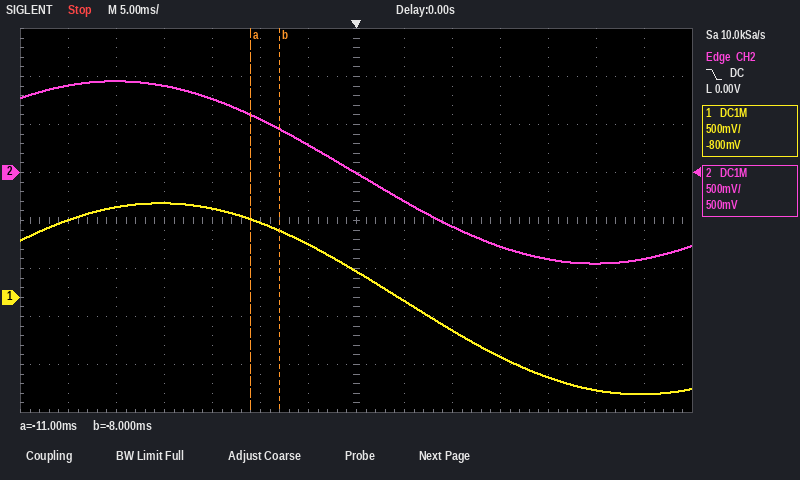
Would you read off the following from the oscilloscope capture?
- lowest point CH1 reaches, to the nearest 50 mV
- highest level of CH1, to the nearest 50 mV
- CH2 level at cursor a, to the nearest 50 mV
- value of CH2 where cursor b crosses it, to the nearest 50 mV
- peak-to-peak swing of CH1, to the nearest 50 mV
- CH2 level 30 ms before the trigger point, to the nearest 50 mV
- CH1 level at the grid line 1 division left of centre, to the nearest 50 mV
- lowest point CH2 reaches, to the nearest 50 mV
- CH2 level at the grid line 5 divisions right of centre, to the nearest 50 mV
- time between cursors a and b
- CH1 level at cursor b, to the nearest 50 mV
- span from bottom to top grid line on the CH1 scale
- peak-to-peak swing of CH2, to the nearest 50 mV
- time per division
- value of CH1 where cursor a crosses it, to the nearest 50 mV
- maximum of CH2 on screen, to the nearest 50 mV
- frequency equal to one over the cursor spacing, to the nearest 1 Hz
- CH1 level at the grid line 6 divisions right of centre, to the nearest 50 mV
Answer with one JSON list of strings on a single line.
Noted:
["-1.00 V", "1.00 V", "600 mV", "450 mV", "2.00 V", "900 mV", "550 mV", "-950 mV", "-950 mV", "3.0 ms", "700 mV", "4 V", "1.90 V", "5 ms", "800 mV", "950 mV", "333 Hz", "-1.00 V"]
